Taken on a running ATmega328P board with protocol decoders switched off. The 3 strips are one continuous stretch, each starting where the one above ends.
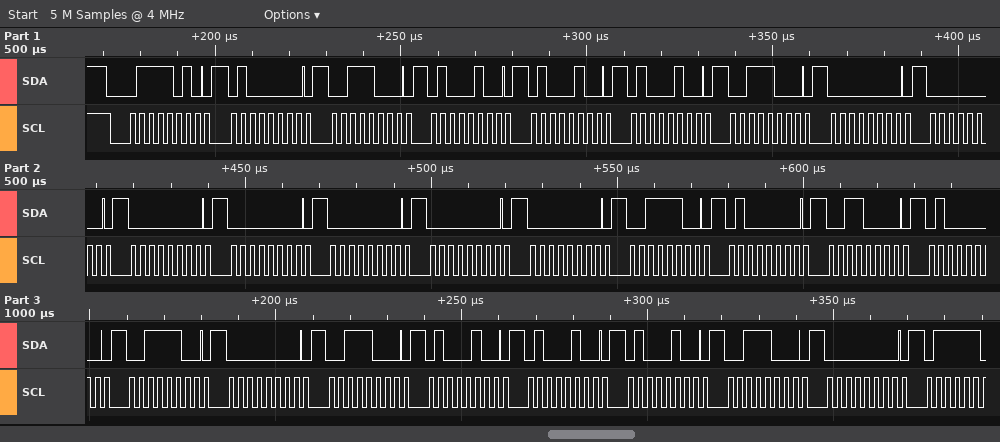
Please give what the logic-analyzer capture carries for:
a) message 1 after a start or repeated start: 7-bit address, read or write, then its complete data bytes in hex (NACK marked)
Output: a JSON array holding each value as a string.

["0x3D write: 40 38 44 44 44 38 00 00 00 00 00 00 00 3C 40 30 40 3C 00 38 44 44 44 38 00"]
